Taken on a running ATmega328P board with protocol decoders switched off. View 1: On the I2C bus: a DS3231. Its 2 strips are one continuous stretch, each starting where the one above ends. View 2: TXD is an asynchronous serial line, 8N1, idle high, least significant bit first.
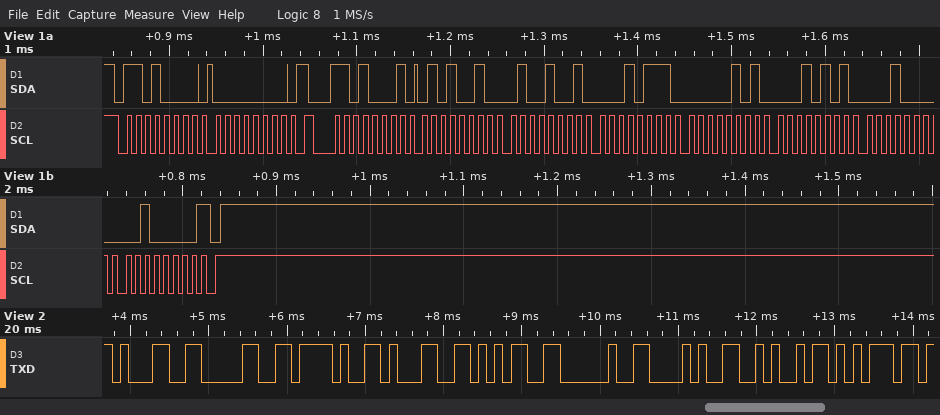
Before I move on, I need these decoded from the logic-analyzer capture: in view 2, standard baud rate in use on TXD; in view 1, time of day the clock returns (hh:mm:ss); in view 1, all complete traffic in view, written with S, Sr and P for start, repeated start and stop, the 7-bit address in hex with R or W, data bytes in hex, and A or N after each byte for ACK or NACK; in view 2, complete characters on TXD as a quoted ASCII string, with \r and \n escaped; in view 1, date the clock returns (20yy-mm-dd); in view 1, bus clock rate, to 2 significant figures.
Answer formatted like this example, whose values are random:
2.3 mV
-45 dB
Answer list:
9600 baud
17:49:52
S 68W A 00 A Sr 68R A 52 A 49 A 17 A 05 A 15 A 10 A 20 N P
"10/15 (Ju"
2020-10-15
100 kHz
